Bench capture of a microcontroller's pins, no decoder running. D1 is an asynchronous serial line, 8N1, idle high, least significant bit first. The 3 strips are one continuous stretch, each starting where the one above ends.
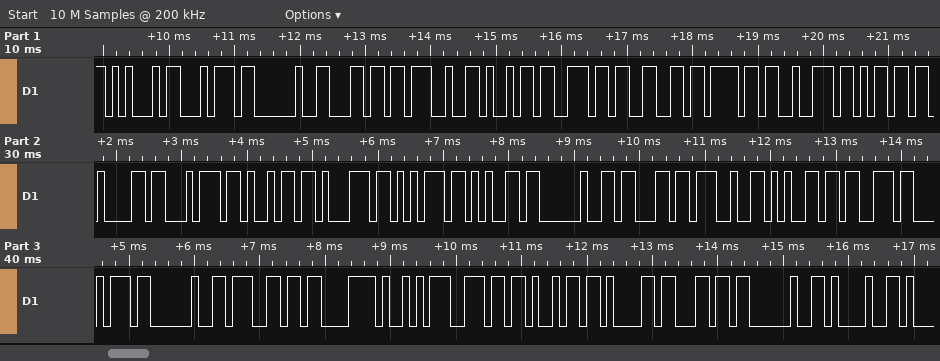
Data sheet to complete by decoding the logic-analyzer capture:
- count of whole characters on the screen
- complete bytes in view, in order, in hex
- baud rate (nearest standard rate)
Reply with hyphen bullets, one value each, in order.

- 33
- 45 74 20 6C 27 69 6E 66 6F 72 6D 61 74 69 71 75 65 20 63 27 65 73 74 20 67 C3 A9 6E 69 61 6C 20 21
- 9600 baud
